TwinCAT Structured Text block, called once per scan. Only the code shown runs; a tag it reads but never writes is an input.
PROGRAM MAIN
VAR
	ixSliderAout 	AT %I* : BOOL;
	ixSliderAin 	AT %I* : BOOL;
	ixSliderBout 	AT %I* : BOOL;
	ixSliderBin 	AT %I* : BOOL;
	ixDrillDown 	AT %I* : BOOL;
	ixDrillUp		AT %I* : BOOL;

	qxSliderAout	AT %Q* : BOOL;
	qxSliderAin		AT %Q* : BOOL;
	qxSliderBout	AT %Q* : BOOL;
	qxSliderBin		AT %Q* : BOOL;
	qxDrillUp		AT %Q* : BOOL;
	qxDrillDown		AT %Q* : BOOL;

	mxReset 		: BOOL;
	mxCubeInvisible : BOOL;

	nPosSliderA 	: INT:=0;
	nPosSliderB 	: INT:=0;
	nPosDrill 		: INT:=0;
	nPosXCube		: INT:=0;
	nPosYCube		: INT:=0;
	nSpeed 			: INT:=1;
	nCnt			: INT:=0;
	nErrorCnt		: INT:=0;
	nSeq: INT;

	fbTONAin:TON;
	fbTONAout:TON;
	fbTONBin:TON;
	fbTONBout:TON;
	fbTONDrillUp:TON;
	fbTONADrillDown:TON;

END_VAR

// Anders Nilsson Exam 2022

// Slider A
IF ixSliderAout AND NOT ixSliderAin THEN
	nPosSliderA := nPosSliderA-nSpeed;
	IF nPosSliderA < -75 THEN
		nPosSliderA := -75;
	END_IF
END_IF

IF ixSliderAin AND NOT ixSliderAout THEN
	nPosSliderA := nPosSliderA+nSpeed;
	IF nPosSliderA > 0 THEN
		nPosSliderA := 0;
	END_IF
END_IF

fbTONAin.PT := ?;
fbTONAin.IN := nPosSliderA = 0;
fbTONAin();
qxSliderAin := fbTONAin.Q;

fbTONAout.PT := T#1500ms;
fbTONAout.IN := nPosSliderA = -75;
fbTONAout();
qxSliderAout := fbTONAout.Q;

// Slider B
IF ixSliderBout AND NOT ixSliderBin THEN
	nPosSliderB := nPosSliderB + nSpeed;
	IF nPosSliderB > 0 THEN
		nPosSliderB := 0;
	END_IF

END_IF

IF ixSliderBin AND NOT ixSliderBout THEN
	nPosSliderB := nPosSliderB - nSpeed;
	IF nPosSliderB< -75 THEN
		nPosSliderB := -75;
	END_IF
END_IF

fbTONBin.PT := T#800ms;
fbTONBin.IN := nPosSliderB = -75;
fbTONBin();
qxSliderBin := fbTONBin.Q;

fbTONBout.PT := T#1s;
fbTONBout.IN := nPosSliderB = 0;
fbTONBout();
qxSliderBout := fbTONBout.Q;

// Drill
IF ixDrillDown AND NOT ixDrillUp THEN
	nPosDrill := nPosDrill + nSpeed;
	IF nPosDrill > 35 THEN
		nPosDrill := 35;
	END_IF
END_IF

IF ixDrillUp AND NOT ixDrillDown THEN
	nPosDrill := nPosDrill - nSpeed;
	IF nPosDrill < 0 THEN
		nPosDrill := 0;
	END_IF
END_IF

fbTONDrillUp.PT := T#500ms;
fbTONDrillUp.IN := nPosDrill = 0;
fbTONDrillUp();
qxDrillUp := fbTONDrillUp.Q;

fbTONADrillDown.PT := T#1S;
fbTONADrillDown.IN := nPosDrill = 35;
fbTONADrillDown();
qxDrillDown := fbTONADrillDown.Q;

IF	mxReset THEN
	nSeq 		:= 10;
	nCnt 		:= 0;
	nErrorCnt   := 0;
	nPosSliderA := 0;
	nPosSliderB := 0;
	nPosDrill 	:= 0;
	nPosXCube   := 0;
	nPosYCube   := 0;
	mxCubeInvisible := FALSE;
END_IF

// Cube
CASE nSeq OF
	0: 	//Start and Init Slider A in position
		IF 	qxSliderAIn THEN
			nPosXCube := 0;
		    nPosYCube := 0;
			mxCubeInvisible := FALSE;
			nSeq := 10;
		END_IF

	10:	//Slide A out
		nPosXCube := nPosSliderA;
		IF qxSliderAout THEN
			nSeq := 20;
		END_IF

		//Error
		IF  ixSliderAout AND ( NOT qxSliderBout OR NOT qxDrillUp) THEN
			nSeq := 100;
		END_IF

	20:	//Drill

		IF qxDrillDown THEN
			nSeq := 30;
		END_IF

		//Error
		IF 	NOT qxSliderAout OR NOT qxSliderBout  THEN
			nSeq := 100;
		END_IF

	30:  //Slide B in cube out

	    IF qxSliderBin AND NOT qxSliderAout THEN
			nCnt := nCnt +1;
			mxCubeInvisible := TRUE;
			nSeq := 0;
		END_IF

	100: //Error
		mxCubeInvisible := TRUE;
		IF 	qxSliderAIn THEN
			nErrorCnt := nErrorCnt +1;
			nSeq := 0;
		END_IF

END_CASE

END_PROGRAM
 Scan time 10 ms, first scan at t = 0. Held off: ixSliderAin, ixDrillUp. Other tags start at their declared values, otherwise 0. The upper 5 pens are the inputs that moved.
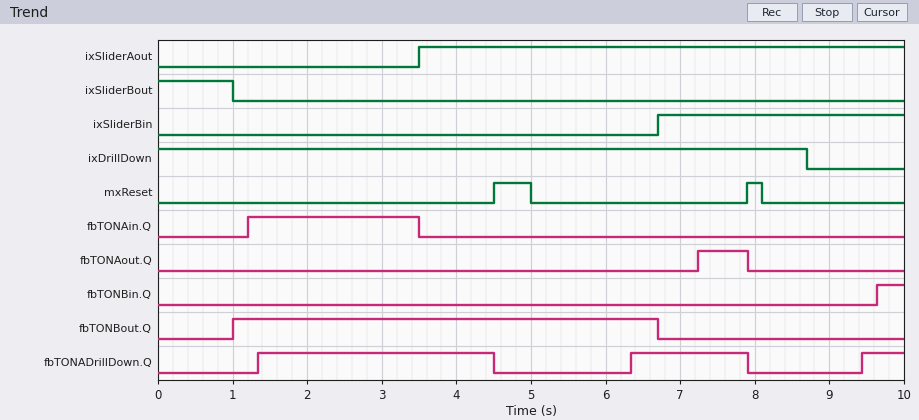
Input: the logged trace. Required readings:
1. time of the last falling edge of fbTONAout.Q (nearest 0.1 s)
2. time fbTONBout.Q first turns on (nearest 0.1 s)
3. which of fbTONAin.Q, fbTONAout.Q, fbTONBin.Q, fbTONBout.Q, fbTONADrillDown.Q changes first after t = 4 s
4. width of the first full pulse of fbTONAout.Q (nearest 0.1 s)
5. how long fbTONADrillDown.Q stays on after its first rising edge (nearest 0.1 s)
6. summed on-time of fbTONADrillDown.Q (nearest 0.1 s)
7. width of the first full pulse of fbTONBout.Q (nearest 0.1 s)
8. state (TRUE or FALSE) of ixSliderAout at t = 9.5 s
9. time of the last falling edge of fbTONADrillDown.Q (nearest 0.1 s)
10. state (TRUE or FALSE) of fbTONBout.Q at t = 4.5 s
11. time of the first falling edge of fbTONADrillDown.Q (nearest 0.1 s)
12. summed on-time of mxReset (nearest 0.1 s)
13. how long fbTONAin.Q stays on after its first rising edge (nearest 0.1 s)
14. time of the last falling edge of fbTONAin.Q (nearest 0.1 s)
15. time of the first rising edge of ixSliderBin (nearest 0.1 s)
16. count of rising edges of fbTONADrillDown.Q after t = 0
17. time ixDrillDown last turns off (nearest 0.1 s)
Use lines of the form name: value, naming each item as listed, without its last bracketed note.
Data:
time of the last falling edge of fbTONAout.Q: 7.9 s
time fbTONBout.Q first turns on: 1.0 s
which of fbTONAin.Q, fbTONAout.Q, fbTONBin.Q, fbTONBout.Q, fbTONADrillDown.Q changes first after t = 4 s: fbTONADrillDown.Q
width of the first full pulse of fbTONAout.Q: 0.7 s
how long fbTONADrillDown.Q stays on after its first rising edge: 3.2 s
summed on-time of fbTONADrillDown.Q: 5.3 s
width of the first full pulse of fbTONBout.Q: 5.7 s
state (TRUE or FALSE) of ixSliderAout at t = 9.5 s: TRUE
time of the last falling edge of fbTONADrillDown.Q: 7.9 s
state (TRUE or FALSE) of fbTONBout.Q at t = 4.5 s: TRUE
time of the first falling edge of fbTONADrillDown.Q: 4.5 s
summed on-time of mxReset: 0.7 s
how long fbTONAin.Q stays on after its first rising edge: 2.3 s
time of the last falling edge of fbTONAin.Q: 3.5 s
time of the first rising edge of ixSliderBin: 6.7 s
count of rising edges of fbTONADrillDown.Q after t = 0: 3
time ixDrillDown last turns off: 8.7 s
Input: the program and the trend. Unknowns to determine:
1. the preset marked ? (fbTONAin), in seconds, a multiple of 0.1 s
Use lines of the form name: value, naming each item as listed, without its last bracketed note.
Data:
the preset marked ? (fbTONAin), in seconds, a multiple of 0.1 s: 1.2 s
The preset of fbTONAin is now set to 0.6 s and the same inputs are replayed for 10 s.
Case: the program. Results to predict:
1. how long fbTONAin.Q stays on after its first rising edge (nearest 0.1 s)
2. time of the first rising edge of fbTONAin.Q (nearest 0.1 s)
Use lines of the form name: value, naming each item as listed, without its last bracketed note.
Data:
how long fbTONAin.Q stays on after its first rising edge: 2.9 s
time of the first rising edge of fbTONAin.Q: 0.6 s
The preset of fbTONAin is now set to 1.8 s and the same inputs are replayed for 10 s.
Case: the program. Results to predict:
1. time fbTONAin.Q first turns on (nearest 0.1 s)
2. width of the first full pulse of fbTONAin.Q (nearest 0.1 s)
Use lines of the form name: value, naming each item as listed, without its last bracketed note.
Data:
time fbTONAin.Q first turns on: 1.8 s
width of the first full pulse of fbTONAin.Q: 1.7 s
